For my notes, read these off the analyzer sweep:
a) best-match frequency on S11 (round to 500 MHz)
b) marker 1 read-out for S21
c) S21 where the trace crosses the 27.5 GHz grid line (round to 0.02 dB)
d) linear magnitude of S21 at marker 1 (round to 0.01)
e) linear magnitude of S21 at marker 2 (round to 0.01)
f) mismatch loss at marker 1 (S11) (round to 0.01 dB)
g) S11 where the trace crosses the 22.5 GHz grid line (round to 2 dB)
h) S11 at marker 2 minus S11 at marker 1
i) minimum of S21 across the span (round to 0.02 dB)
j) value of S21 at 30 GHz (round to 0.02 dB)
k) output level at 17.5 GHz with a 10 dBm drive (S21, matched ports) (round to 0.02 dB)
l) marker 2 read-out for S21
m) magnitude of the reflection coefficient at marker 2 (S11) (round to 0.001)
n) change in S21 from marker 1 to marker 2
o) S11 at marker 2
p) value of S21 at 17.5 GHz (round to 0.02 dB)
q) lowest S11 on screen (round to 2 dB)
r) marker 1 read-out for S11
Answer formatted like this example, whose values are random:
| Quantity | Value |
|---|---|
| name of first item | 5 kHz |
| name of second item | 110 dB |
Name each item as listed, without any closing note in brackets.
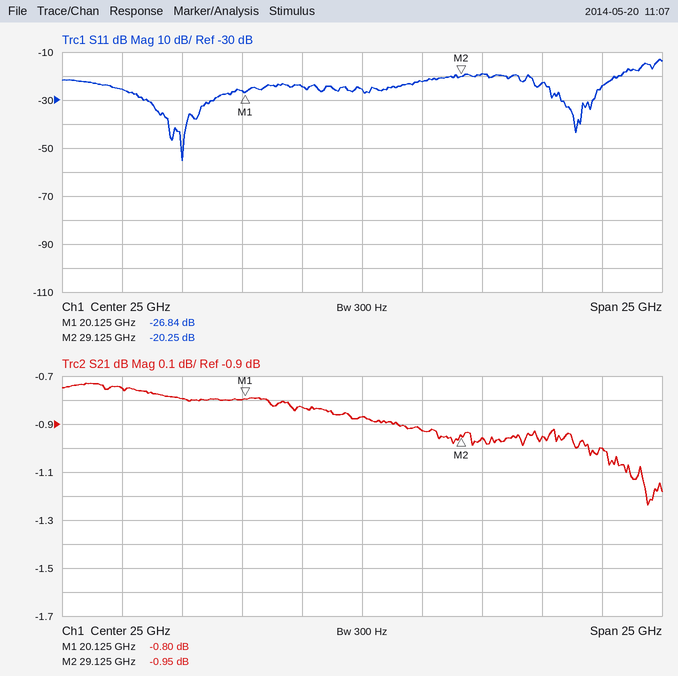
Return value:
| Quantity | Value |
|---|---|
| best-match frequency on S11 | 17.5 GHz |
| marker 1 read-out for S21 | -0.80 dB |
| S21 where the trace crosses the 27.5 GHz grid line | -0.92 dB |
| linear magnitude of S21 at marker 1 | 0.91 |
| linear magnitude of S21 at marker 2 | 0.90 |
| mismatch loss at marker 1 (S11) | 0.01 dB |
| S11 where the trace crosses the 22.5 GHz grid line | -24 dB |
| S11 at marker 2 minus S11 at marker 1 | 6.59 dB |
| minimum of S21 across the span | -1.24 dB |
| value of S21 at 30 GHz | -0.96 dB |
| output level at 17.5 GHz with a 10 dBm drive (S21, matched ports) | 9.20 dBm |
| marker 2 read-out for S21 | -0.95 dB |
| magnitude of the reflection coefficient at marker 2 (S11) | 0.097 |
| change in S21 from marker 1 to marker 2 | -0.15 dB |
| S11 at marker 2 | -20.25 dB |
| value of S21 at 17.5 GHz | -0.80 dB |
| lowest S11 on screen | -56 dB |
| marker 1 read-out for S11 | -26.84 dB |
